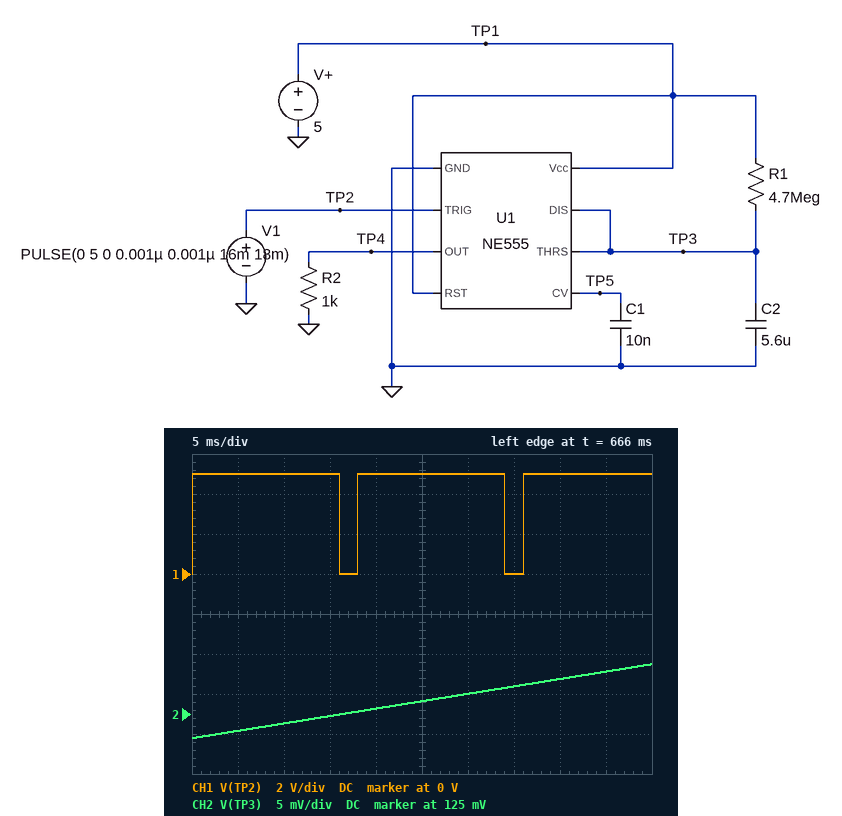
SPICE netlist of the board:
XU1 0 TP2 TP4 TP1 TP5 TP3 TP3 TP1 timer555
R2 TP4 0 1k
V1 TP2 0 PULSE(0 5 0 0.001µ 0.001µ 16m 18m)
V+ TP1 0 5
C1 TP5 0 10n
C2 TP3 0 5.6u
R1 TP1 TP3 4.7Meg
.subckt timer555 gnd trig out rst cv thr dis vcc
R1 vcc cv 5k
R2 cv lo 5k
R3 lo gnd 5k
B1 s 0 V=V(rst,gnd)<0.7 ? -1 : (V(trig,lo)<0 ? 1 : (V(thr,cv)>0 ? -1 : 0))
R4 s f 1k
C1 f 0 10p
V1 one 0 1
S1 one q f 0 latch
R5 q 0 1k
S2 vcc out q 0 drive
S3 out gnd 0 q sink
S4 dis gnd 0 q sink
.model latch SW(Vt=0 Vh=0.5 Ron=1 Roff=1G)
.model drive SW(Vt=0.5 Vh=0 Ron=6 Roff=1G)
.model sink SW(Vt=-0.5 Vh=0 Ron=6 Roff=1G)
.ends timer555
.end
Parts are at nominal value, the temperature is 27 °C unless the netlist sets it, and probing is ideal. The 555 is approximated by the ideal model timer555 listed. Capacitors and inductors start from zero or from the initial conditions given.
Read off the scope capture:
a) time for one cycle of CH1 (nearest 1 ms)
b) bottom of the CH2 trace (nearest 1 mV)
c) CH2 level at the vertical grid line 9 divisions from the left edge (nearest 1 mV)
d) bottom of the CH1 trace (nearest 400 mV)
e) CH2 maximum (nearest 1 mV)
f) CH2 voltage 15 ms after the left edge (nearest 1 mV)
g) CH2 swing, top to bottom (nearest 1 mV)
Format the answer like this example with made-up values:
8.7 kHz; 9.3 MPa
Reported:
18 ms; 122 mV; 130 mV; 0 V; 131 mV; 125 mV; 9 mV
